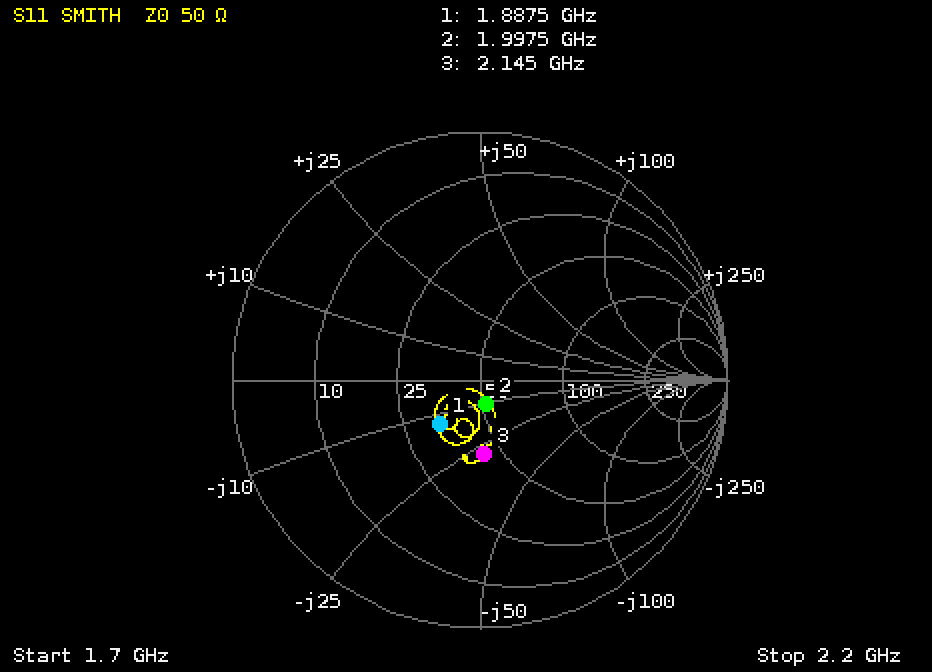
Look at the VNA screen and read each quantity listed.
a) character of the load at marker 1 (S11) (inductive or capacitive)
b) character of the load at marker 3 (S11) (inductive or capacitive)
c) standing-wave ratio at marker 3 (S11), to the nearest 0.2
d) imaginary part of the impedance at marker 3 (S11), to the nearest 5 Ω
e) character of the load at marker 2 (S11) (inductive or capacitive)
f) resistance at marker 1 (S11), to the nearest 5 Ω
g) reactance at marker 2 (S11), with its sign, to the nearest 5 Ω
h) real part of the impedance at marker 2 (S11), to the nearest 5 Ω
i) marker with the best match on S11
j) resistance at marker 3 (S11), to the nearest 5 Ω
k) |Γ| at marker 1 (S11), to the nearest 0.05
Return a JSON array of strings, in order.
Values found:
["capacitive", "capacitive", "1.8", "-30 Ω", "capacitive", "35 Ω", "-10 Ω", "50 Ω", "marker 2", "45 Ω", "0.25"]
